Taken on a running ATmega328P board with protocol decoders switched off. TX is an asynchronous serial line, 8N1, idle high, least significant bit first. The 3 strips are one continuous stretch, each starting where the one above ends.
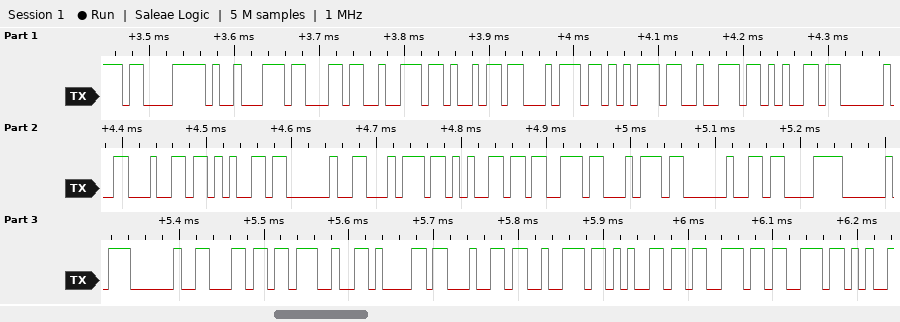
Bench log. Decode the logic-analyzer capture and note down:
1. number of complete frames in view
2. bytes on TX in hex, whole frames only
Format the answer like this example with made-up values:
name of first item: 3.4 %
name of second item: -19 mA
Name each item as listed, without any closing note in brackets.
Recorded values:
number of complete frames in view: 29
bytes on TX in hex, whole frames only: 0xC3 0x89 0x63 0x72 0x69 0x74 0x75 0x72 0x65 0x20 0x64 0x65 0x20 0x74 0x65 0x73 0x74 0x20 0xC3 0xA0 0x20 0x6C 0x27 0x61 0x64 0x72 0x65 0x73 0x73
